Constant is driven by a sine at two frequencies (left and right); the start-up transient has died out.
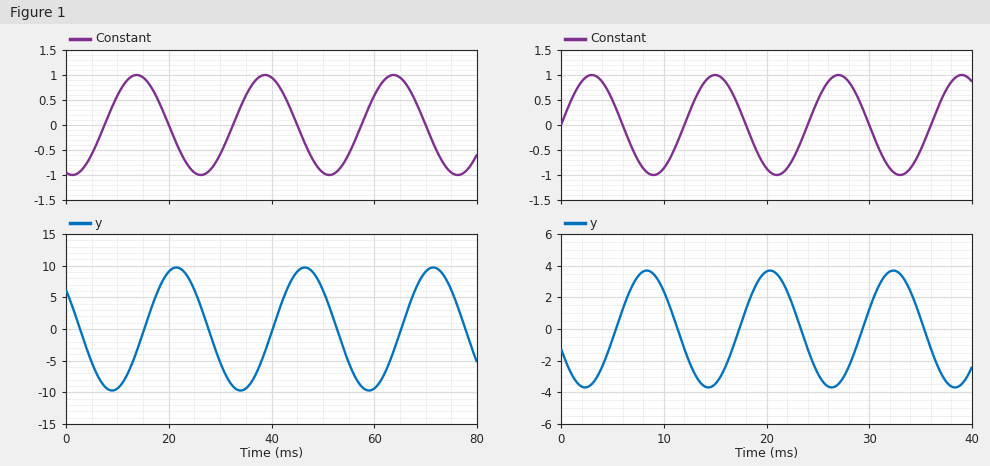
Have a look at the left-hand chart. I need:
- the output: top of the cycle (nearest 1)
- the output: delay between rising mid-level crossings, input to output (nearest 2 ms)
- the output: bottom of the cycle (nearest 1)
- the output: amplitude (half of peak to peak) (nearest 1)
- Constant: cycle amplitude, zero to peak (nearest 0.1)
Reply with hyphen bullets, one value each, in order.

- 10
- 8 ms
- -10
- 10
- 1.0
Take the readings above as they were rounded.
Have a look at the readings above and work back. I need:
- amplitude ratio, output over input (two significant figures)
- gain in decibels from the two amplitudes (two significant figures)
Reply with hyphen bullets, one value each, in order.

- 10
- 20 dB
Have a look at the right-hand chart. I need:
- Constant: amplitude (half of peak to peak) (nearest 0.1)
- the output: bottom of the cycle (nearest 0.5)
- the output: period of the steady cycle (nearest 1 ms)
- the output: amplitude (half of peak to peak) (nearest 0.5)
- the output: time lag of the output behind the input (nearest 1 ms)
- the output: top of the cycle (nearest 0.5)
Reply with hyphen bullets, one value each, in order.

- 1.0
- -3.5
- 12 ms
- 3.5
- 5 ms
- 3.5
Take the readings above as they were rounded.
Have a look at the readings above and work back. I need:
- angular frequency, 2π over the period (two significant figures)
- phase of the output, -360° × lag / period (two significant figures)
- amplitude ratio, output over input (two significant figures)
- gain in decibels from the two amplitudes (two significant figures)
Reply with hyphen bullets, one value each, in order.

- 0.52 rad/ms
- -150°
- 3.5
- 11 dB
